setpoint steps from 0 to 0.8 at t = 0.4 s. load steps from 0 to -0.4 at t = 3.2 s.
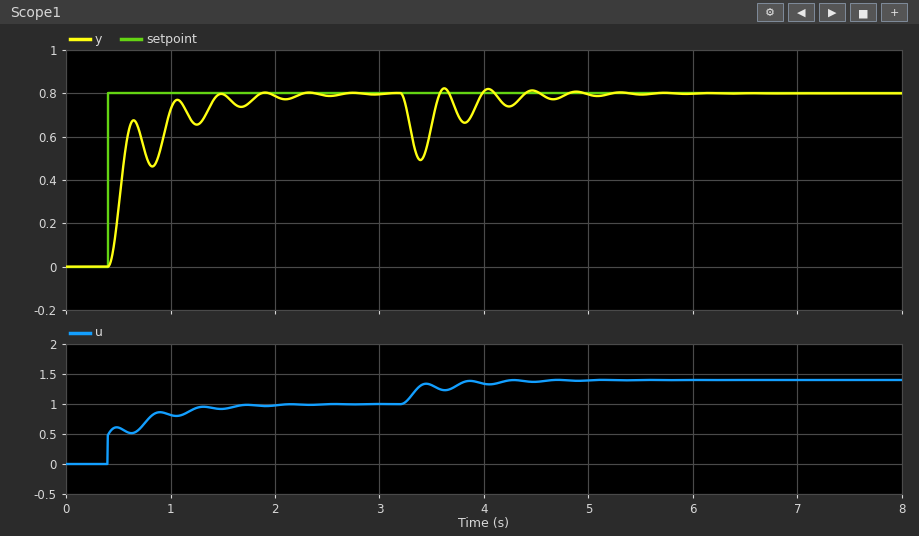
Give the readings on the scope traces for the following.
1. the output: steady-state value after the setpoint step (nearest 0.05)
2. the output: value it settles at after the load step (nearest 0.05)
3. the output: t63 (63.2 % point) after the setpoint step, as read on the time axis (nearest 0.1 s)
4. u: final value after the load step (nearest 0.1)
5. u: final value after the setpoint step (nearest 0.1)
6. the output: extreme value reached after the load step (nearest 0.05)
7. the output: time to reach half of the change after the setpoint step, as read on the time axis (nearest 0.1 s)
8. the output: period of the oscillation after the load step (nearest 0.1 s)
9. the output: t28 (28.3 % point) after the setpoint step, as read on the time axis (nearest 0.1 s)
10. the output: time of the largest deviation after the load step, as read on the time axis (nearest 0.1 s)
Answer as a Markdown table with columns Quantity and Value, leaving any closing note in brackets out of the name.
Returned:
| Quantity | Value |
|---|---|
| the output: steady-state value after the setpoint step | 0.80 |
| the output: value it settles at after the load step | 0.80 |
| the output: t63 (63.2 % point) after the setpoint step, as read on the time axis | 0.6 s |
| u: final value after the load step | 1.4 |
| u: final value after the setpoint step | 1.0 |
| the output: extreme value reached after the load step | 0.50 |
| the output: time to reach half of the change after the setpoint step, as read on the time axis | 0.5 s |
| the output: period of the oscillation after the load step | 0.4 s |
| the output: t28 (28.3 % point) after the setpoint step, as read on the time axis | 0.5 s |
| the output: time of the largest deviation after the load step, as read on the time axis | 3.4 s |
